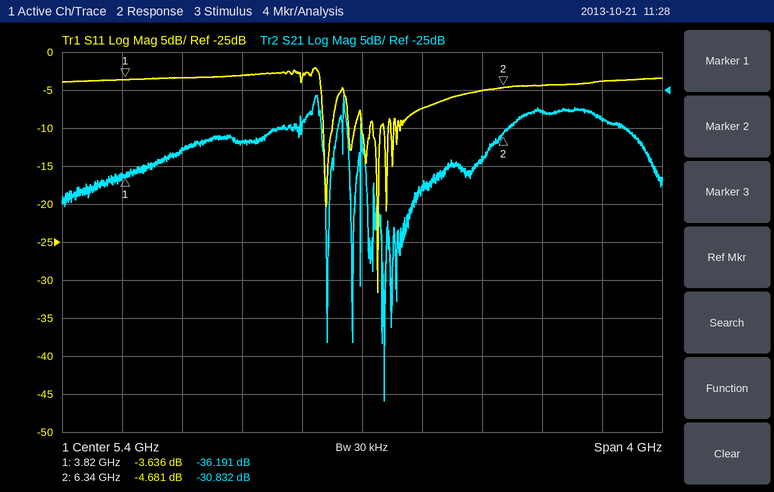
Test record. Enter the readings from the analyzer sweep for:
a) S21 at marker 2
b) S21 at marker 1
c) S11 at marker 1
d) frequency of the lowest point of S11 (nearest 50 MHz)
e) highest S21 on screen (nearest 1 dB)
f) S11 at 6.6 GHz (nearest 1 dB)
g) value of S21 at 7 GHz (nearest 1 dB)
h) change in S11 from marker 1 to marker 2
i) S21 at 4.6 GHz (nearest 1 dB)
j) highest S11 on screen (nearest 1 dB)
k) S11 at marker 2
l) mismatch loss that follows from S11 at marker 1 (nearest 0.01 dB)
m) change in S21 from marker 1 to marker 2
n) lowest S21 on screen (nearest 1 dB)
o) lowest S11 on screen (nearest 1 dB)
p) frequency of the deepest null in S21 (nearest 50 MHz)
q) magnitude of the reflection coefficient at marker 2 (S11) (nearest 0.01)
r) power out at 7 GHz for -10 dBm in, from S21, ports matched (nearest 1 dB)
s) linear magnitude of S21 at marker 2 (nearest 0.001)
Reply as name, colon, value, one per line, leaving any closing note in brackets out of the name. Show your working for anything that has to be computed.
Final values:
S21 at marker 2: -30.832 dB
S21 at marker 1: -36.191 dB
S11 at marker 1: -3.636 dB
frequency of the lowest point of S11: 5.50 GHz
highest S21 on screen: -26 dB
S11 at 6.6 GHz: -4 dB
value of S21 at 7 GHz: -29 dB
change in S11 from marker 1 to marker 2: -4.681 − (-3.636) = -1.045 dB
S21 at 4.6 GHz: -32 dB
highest S11 on screen: -2 dB
S11 at marker 2: -4.681 dB
mismatch loss that follows from S11 at marker 1: −10 log10(1 − 10^(-3.636/10)) ≈ 2.46 dB
change in S21 from marker 1 to marker 2: -30.832 − (-36.191) = 5.359 dB
lowest S21 on screen: -66 dB
lowest S11 on screen: -32 dB
frequency of the deepest null in S21: 5.55 GHz
magnitude of the reflection coefficient at marker 2 (S11): 10^(-4.681/20) ≈ 0.58
power out at 7 GHz for -10 dBm in, from S21, ports matched: -10 dBm + (-29 dB) = -39 dBm
linear magnitude of S21 at marker 2: 10^(-30.832/20) ≈ 0.029
